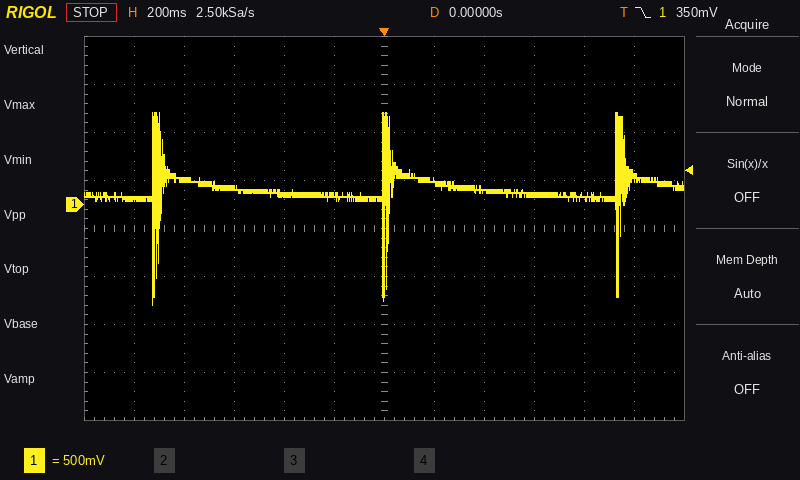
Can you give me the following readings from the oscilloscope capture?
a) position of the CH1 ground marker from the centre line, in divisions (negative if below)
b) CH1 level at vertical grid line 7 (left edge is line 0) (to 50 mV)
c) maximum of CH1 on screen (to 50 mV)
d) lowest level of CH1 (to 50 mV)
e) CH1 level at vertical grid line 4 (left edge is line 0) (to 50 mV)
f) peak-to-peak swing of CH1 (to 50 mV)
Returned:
+0.5 div
250 mV
950 mV
-1.05 V
100 mV
2.00 V
